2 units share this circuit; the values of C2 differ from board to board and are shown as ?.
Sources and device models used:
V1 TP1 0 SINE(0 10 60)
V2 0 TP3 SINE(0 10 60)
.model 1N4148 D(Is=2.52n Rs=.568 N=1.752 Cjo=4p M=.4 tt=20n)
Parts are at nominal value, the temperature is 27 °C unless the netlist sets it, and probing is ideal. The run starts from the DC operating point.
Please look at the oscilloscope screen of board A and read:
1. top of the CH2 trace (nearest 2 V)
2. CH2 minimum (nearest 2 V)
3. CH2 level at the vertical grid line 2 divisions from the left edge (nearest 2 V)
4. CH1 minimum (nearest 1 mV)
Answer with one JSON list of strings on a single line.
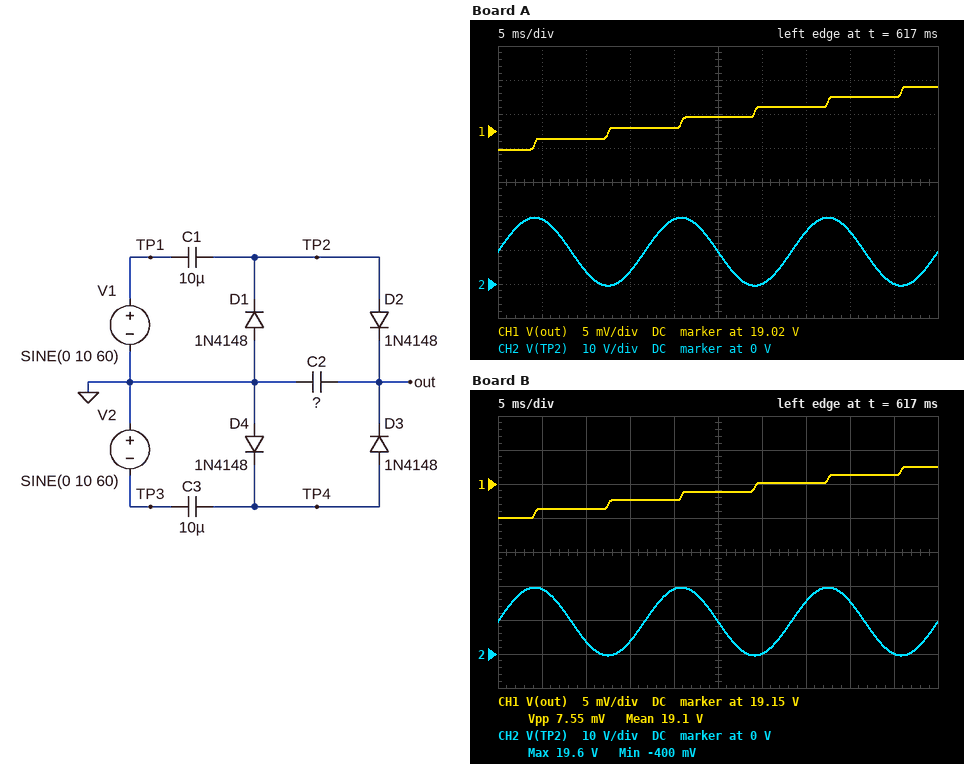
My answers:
["20 V", "0 V", "4 V", "19.012 V"]
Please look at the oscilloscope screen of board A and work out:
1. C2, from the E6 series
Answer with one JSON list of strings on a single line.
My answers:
["33 µF"]
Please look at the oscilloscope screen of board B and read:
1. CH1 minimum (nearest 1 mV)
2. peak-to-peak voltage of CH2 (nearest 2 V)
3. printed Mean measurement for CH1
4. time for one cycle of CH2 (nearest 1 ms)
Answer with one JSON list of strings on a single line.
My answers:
["19.145 V", "20 V", "19.1 V", "17 ms"]
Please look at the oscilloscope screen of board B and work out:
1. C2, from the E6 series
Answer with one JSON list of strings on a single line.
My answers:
["6.8 µF"]
